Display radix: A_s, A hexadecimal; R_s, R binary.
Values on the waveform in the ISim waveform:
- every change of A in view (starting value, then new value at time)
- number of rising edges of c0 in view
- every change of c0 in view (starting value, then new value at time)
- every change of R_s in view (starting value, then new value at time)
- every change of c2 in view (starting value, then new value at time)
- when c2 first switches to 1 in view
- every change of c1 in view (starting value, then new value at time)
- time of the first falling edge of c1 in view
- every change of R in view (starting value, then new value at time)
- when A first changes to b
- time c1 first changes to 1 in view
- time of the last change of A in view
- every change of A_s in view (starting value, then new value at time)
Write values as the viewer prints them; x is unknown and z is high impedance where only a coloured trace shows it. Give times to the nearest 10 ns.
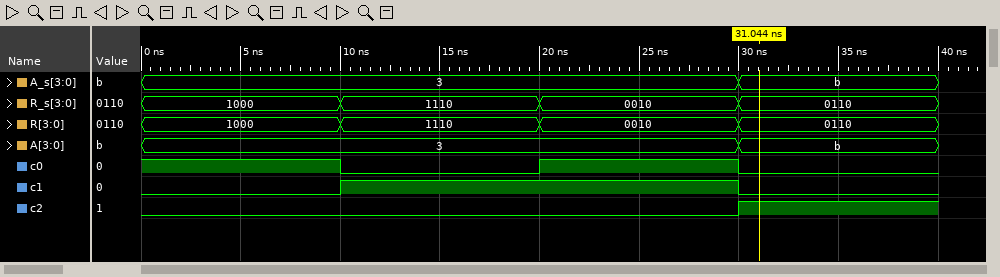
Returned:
3, b at 30 ns
1
1, 0 at 10 ns, 1 at 20 ns, 0 at 30 ns
1000, 1110 at 10 ns, 0010 at 20 ns, 0110 at 30 ns
0, 1 at 30 ns
30 ns
0, 1 at 10 ns, 0 at 30 ns
30 ns
1000, 1110 at 10 ns, 0010 at 20 ns, 0110 at 30 ns
30 ns
10 ns
30 ns
3, b at 30 ns
